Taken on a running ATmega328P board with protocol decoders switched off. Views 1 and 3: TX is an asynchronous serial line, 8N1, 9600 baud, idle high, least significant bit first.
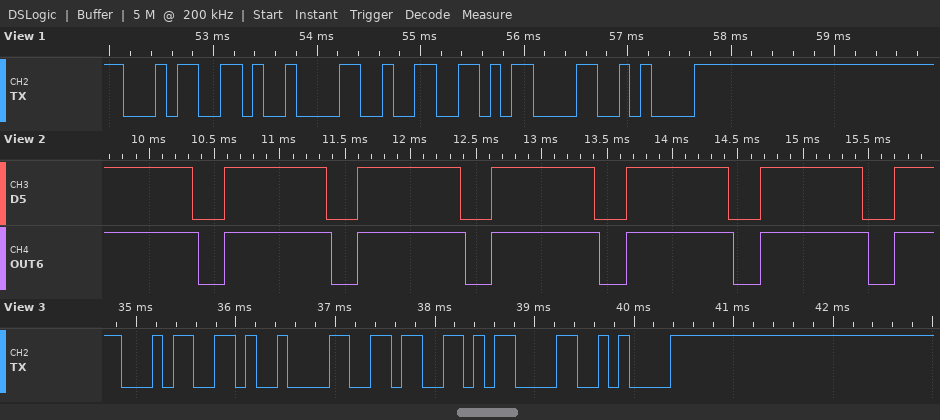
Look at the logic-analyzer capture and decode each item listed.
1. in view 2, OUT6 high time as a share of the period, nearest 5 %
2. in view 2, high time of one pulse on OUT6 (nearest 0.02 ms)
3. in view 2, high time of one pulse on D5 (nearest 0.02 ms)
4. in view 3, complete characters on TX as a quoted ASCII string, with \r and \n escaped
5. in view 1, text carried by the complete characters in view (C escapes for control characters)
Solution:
80 %
0.82 ms
0.78 ms
"4\t6\r\n"
"4\t2\r\n"
